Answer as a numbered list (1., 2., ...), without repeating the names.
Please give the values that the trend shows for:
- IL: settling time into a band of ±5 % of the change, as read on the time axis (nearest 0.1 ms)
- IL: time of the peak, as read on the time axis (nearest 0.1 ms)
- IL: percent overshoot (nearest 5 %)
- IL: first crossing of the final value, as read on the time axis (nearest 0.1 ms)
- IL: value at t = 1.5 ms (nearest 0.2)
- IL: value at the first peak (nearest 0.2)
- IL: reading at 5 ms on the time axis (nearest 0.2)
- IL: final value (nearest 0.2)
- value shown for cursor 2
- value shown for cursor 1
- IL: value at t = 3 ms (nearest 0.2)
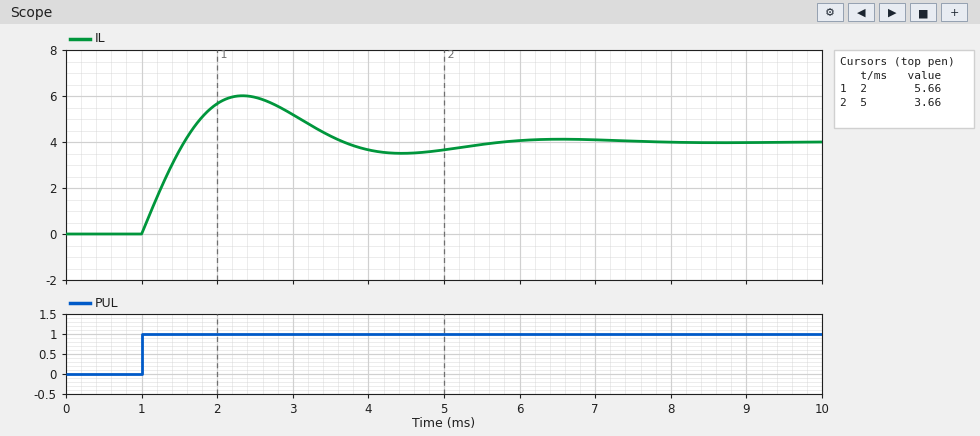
1. 5.3 ms
2. 2.3 ms
3. 50 %
4. 1.6 ms
5. 3.6
6. 6.0
7. 3.6
8. 4.0
9. 3.66
10. 5.66
11. 5.2
